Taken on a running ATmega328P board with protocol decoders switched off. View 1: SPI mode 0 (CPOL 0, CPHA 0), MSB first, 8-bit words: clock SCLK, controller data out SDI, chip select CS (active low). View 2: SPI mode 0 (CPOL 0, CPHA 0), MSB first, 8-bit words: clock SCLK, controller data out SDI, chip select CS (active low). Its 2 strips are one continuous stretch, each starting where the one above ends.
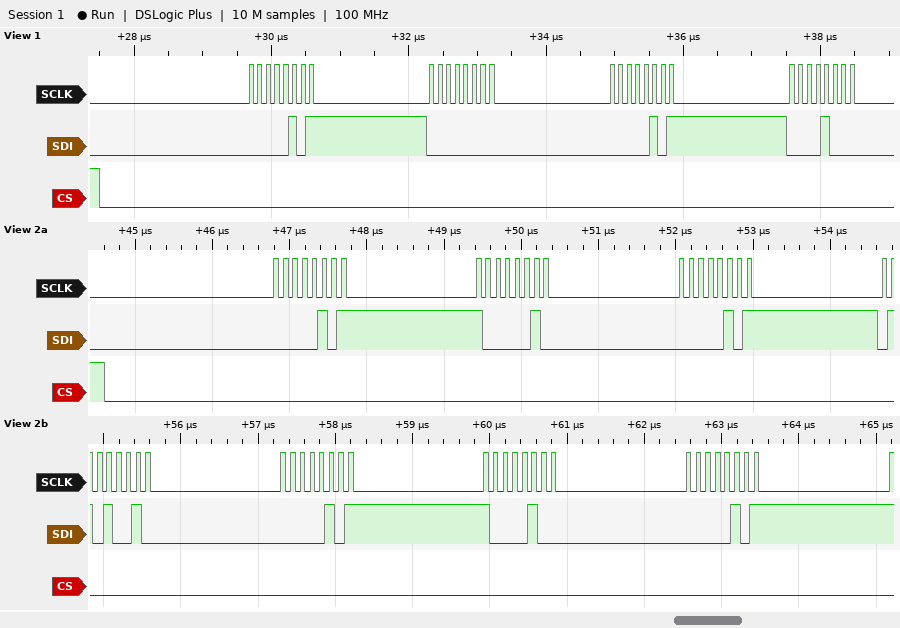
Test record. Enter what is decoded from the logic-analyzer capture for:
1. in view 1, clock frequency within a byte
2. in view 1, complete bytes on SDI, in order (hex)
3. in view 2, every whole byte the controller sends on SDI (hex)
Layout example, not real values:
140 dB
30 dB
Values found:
8 MHz
0x05 0x00 0x05 0x08
05 82 05 52 05 84 05
